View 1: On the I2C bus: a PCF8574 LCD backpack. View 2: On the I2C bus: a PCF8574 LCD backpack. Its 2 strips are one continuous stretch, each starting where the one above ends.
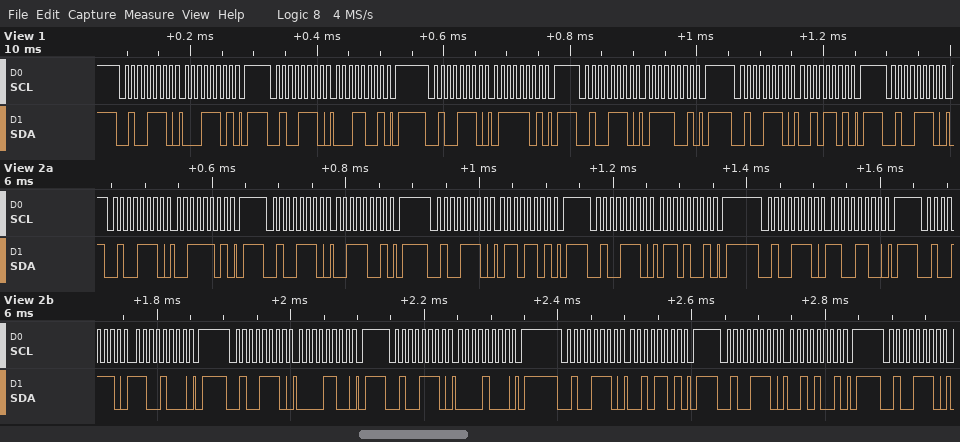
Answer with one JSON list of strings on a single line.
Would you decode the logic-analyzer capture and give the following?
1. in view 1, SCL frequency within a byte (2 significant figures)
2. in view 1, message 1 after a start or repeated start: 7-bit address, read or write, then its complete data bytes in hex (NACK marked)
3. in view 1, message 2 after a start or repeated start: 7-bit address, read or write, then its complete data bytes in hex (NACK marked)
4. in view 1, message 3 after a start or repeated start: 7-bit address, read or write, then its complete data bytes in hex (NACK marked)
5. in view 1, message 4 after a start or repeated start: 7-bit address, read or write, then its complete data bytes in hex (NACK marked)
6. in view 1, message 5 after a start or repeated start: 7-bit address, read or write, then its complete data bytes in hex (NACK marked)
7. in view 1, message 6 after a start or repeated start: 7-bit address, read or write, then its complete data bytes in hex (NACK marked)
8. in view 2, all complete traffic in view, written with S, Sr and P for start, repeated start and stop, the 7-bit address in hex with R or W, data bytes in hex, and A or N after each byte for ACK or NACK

["100 kHz", "0x27 write: 1D", "0x27 write: 19", "0x27 write: 7D", "0x27 write: 79", "0x27 write: 2D", "0x27 write", "S 27W A 3D A P S 27W A 39 A P S 27W A 6D A P S 27W A 69 A P S 27W A CC A P S 27W A C8 A P S 27W A 0C A P S 27W A 08 A P S 27W A 2D A P S 27W A 29 A P S 27W A"]
